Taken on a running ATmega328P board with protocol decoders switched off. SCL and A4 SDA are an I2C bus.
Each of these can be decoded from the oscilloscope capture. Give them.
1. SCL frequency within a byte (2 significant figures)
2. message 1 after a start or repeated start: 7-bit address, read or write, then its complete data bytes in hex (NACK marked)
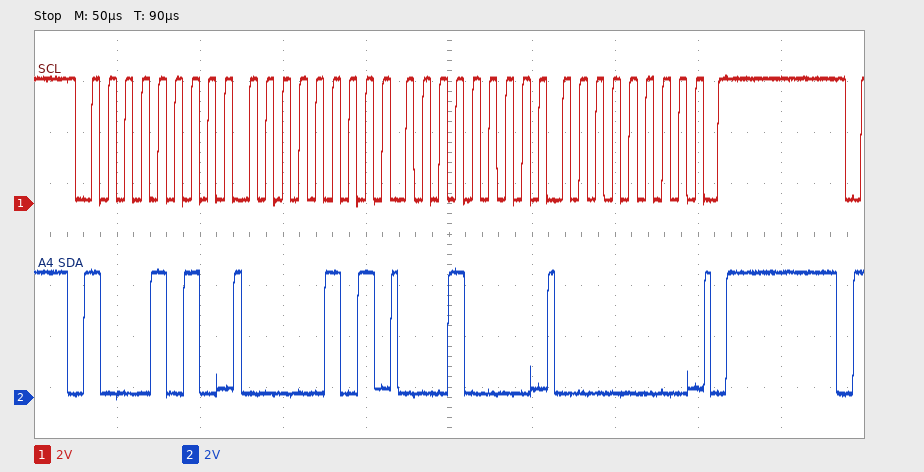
100 kHz
0x45 write: 05 10 00
